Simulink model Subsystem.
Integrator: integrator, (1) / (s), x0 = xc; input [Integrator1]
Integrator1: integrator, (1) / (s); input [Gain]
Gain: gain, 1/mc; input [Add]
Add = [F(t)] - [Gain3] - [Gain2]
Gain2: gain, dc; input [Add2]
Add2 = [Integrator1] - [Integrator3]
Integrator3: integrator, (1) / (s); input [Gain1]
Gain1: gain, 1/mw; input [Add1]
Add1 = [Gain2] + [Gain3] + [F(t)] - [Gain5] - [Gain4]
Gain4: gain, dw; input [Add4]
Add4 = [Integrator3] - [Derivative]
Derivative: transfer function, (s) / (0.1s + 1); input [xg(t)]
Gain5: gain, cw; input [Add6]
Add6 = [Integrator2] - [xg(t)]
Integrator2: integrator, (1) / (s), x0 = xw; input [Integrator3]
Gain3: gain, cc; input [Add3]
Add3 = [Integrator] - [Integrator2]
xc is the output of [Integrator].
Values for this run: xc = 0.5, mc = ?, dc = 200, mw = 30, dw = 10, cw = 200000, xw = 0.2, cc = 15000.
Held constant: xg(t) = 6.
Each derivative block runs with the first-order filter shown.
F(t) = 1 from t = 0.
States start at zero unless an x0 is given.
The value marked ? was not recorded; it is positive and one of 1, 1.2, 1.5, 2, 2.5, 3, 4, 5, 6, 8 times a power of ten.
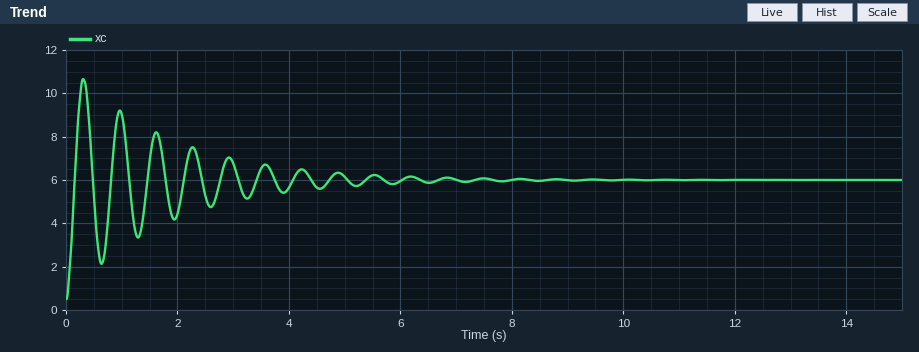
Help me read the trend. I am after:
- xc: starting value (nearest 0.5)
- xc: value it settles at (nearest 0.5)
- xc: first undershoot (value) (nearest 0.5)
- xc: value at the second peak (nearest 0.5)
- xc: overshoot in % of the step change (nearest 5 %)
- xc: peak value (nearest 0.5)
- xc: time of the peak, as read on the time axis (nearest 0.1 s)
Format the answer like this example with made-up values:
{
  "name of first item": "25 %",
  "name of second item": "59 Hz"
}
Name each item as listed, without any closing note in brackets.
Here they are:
{
  "xc: starting value": "0.5",
  "xc: value it settles at": "6.0",
  "xc: first undershoot (value)": "2.0",
  "xc: value at the second peak": "9.0",
  "xc: overshoot in % of the step change": "85 %",
  "xc: peak value": "10.5",
  "xc: time of the peak, as read on the time axis": "0.3 s"
}
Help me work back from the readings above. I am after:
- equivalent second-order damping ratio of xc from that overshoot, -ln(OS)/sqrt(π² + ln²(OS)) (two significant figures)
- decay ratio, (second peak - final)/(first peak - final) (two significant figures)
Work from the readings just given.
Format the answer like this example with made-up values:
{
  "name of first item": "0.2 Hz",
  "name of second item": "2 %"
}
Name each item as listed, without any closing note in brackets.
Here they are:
{
  "equivalent second-order damping ratio of xc from that overshoot, -ln(OS)/sqrt(π² + ln²(OS))": "0.052",
  "decay ratio, (second peak - final)/(first peak - final)": "0.67"
}
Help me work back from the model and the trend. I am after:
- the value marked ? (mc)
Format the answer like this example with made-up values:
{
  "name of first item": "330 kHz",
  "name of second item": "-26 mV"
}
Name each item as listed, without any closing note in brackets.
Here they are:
{
  "the value marked ?": "150"
}
